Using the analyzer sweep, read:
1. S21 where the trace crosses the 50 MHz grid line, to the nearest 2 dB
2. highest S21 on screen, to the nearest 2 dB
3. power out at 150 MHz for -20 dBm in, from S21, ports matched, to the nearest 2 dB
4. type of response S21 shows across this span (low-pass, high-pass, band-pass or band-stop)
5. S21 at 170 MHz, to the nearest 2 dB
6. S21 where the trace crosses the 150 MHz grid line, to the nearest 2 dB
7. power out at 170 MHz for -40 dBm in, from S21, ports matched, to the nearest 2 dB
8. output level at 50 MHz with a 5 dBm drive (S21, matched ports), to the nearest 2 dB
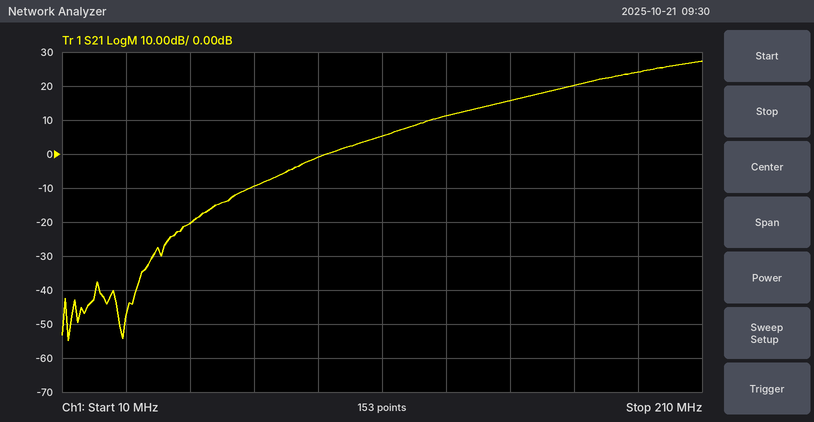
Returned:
-20 dB
28 dB
-4 dBm
high-pass
20 dB
16 dB
-20 dBm
-16 dBm
